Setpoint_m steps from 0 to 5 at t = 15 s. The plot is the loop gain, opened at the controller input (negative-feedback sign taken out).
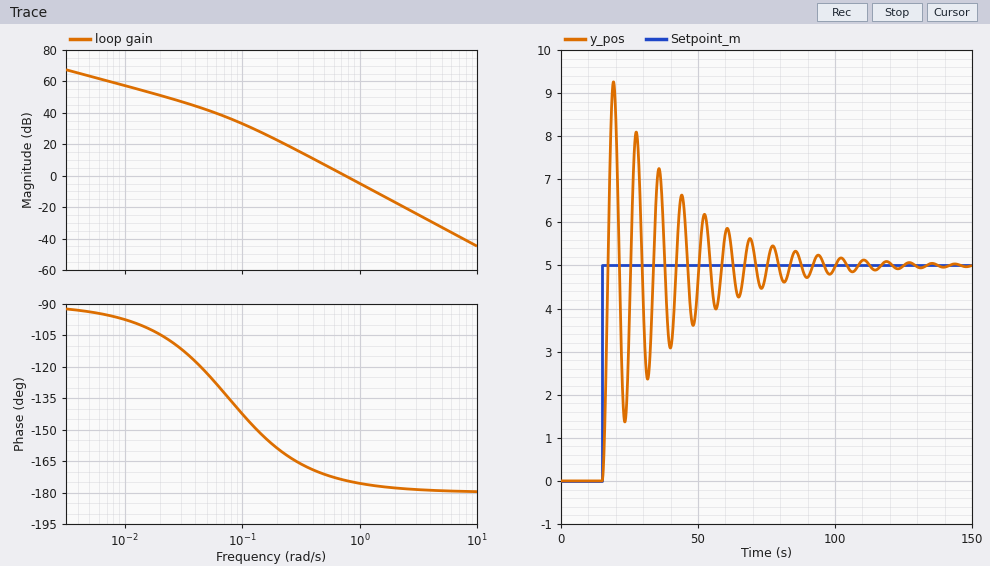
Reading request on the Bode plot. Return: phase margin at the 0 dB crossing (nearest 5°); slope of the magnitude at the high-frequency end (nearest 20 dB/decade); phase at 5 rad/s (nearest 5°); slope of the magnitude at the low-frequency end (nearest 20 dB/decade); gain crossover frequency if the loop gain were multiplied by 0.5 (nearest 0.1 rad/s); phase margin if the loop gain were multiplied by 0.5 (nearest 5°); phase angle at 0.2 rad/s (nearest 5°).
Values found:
5°
-40 dB/decade
-180°
-20 dB/decade
0.5 rad/s
10°
-160°
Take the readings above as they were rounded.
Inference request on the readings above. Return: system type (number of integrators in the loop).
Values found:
1
